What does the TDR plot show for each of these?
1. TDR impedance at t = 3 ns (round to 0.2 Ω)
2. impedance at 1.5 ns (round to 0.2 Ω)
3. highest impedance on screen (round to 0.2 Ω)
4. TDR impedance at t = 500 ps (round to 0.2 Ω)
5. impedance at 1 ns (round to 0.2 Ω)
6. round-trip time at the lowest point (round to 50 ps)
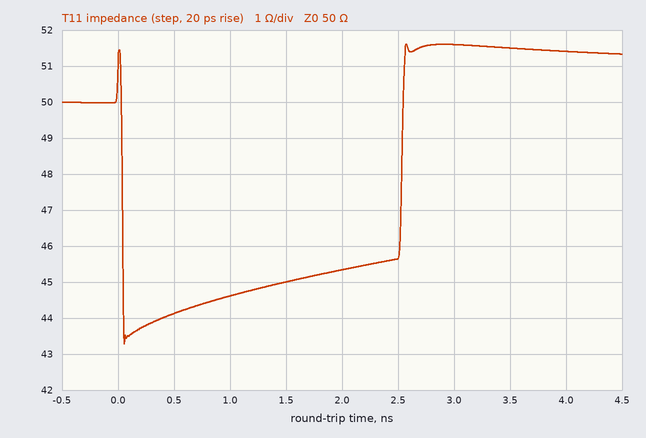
51.6 Ω
45.0 Ω
51.6 Ω
44.2 Ω
44.6 Ω
50 ps
